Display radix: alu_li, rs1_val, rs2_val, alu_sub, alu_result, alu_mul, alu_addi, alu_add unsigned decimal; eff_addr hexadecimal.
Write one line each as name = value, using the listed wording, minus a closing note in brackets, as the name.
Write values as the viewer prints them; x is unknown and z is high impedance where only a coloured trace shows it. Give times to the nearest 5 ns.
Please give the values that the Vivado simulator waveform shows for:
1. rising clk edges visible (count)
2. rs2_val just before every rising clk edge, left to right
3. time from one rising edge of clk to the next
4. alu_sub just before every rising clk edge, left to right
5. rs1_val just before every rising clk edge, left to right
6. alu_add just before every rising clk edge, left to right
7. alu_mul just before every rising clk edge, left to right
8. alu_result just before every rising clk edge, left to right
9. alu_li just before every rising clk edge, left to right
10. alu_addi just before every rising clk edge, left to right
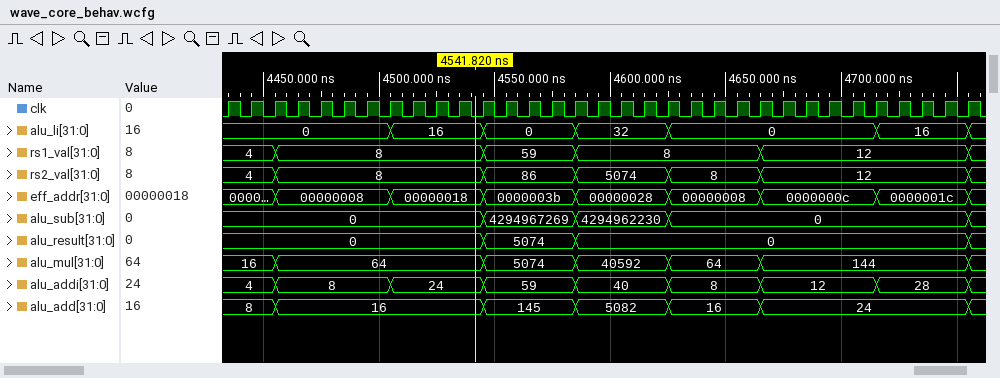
rising clk edges visible = 33
rs2_val just before every rising clk edge, left to right = 4, 4, 4, 8, 8, 8, 8, 8, 8, 8, 8, 8, 86, 86, 86, 86, 5074, 5074, 5074, 5074, 8, 8, 8, 8, 12, 12, 12, 12, 12, 12, 12, 12, 12
time from one rising edge of clk to the next = 10 ns
alu_sub just before every rising clk edge, left to right = 0, 0, 0, 0, 0, 0, 0, 0, 0, 0, 0, 0, 4294967269, 4294967269, 4294967269, 4294967269, 4294962230, 4294962230, 4294962230, 4294962230, 0, 0, 0, 0, 0, 0, 0, 0, 0, 0, 0, 0, 0
rs1_val just before every rising clk edge, left to right = 4, 4, 4, 8, 8, 8, 8, 8, 8, 8, 8, 8, 59, 59, 59, 59, 8, 8, 8, 8, 8, 8, 8, 8, 12, 12, 12, 12, 12, 12, 12, 12, 12
alu_add just before every rising clk edge, left to right = 8, 8, 8, 16, 16, 16, 16, 16, 16, 16, 16, 16, 145, 145, 145, 145, 5082, 5082, 5082, 5082, 16, 16, 16, 16, 24, 24, 24, 24, 24, 24, 24, 24, 24
alu_mul just before every rising clk edge, left to right = 16, 16, 16, 64, 64, 64, 64, 64, 64, 64, 64, 64, 5074, 5074, 5074, 5074, 40592, 40592, 40592, 40592, 64, 64, 64, 64, 144, 144, 144, 144, 144, 144, 144, 144, 144
alu_result just before every rising clk edge, left to right = 0, 0, 0, 0, 0, 0, 0, 0, 0, 0, 0, 0, 5074, 5074, 5074, 5074, 0, 0, 0, 0, 0, 0, 0, 0, 0, 0, 0, 0, 0, 0, 0, 0, 0
alu_li just before every rising clk edge, left to right = 0, 0, 0, 0, 0, 0, 0, 0, 16, 16, 16, 16, 0, 0, 0, 0, 32, 32, 32, 32, 0, 0, 0, 0, 0, 0, 0, 0, 0, 16, 16, 16, 16
alu_addi just before every rising clk edge, left to right = 4, 4, 4, 8, 8, 8, 8, 8, 24, 24, 24, 24, 59, 59, 59, 59, 40, 40, 40, 40, 8, 8, 8, 8, 12, 12, 12, 12, 12, 28, 28, 28, 28
